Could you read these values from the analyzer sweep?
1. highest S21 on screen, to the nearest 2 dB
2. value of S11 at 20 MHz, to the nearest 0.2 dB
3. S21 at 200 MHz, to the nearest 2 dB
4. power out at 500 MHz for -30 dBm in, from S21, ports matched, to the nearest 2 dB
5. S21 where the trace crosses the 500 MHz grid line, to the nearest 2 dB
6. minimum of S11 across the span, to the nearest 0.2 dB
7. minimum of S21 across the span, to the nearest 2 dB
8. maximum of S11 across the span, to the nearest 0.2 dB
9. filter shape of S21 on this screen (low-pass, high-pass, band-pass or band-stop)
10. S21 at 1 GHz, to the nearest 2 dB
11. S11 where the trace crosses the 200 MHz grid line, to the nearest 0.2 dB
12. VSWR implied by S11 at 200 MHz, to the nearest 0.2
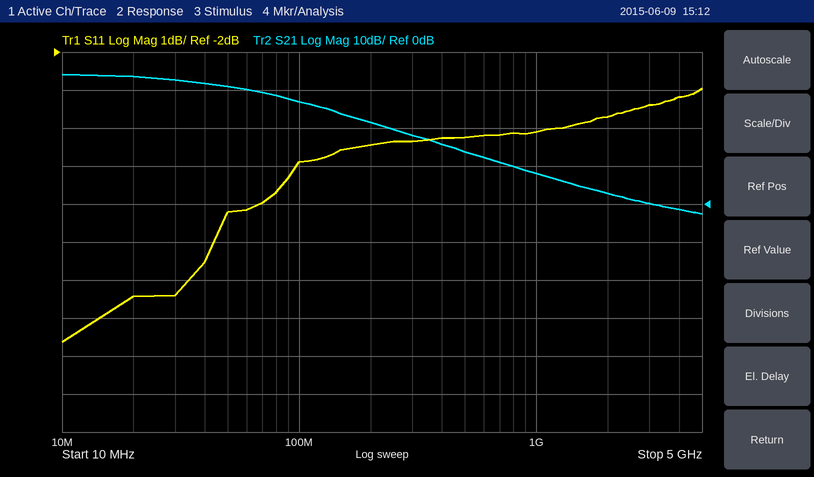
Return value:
34 dB
-8.4 dB
22 dB
-16 dBm
14 dB
-9.6 dB
-2 dB
-3.0 dB
low-pass
8 dB
-4.4 dB
4.0
